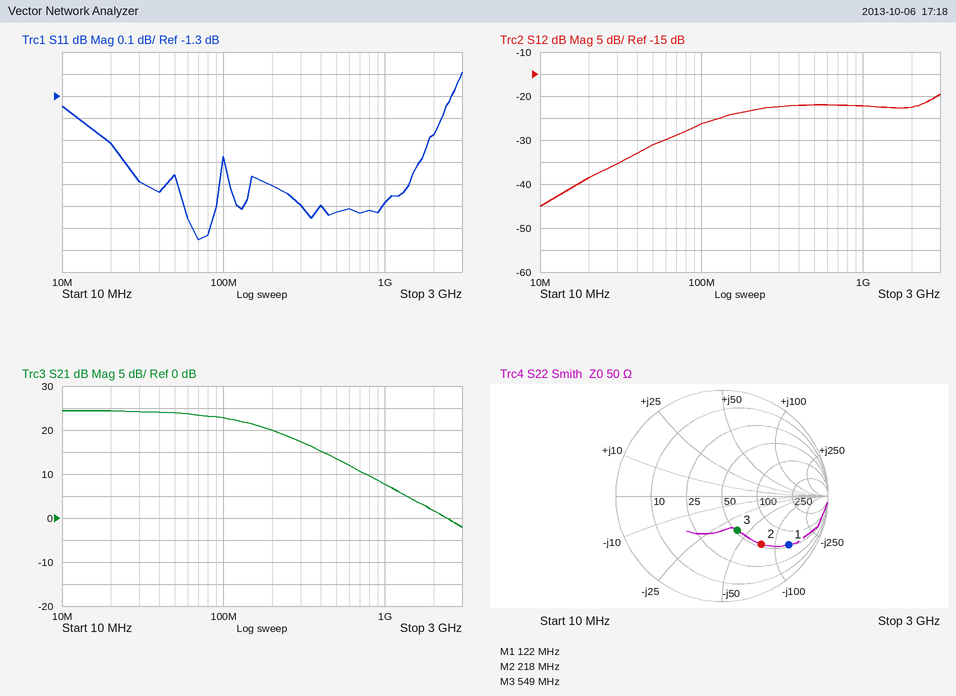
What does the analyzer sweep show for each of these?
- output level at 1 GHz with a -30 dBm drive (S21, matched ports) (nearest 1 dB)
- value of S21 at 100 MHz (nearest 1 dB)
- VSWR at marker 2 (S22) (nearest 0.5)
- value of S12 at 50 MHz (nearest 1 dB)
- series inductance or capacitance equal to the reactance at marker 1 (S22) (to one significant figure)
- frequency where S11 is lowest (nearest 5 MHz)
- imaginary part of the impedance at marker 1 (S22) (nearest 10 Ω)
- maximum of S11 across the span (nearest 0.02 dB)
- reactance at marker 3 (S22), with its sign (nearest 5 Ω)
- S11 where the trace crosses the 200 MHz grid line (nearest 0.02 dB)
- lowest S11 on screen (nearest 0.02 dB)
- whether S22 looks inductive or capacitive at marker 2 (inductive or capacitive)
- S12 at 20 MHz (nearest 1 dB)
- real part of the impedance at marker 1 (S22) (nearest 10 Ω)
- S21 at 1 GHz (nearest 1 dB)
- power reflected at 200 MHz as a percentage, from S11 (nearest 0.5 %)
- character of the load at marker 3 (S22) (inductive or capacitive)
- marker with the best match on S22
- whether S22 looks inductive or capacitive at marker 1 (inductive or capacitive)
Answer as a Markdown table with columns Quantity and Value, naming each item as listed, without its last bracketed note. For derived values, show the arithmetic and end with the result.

| Quantity | Value |
|---|---|
| output level at 1 GHz with a -30 dBm drive (S21, matched ports) | -30 dBm + (8 dB) = -22 dBm |
| value of S21 at 100 MHz | 23 dB |
| VSWR at marker 2 (S22) | 4.0 |
| value of S12 at 50 MHz | -31 dB |
| series inductance or capacitance equal to the reactance at marker 1 (S22) | C = 1/(2π × 122 MHz × 130 Ω) ≈ 10 pF |
| frequency where S11 is lowest | 70 MHz |
| imaginary part of the impedance at marker 1 (S22) | -130 Ω |
| maximum of S11 across the span | -1.20 dB |
| reactance at marker 3 (S22), with its sign | -40 Ω |
| S11 where the trace crosses the 200 MHz grid line | -1.70 dB |
| lowest S11 on screen | -1.96 dB |
| whether S22 looks inductive or capacitive at marker 2 | capacitive |
| S12 at 20 MHz | -39 dB |
| real part of the impedance at marker 1 (S22) | 60 Ω |
| S21 at 1 GHz | 8 dB |
| power reflected at 200 MHz as a percentage, from S11 | 10^(-1.7/10) ≈ 67.6 %, so 67.5 % to the nearest 0.5 % |
| character of the load at marker 3 (S22) | capacitive |
| marker with the best match on S22 | marker 3 |
| whether S22 looks inductive or capacitive at marker 1 | capacitive |
